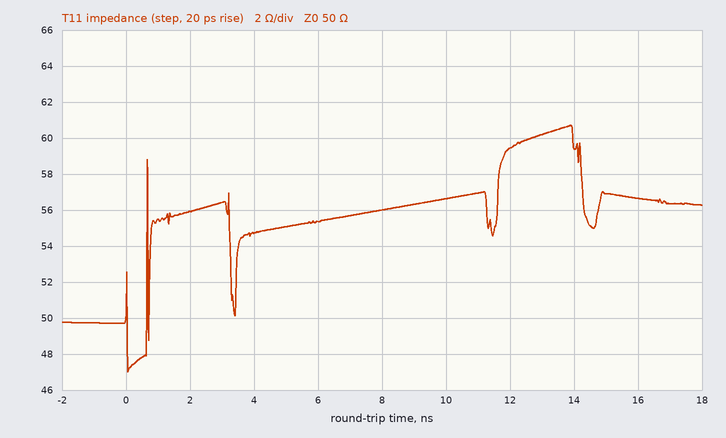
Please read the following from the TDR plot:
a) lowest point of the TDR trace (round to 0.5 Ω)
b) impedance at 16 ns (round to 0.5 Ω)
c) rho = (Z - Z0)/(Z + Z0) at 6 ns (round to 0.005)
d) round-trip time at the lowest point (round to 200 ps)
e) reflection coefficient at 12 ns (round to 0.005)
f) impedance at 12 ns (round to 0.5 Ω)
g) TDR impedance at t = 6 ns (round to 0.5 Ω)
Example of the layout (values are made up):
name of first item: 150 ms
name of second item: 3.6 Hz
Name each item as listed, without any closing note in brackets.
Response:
lowest point of the TDR trace: 47.0 Ω
impedance at 16 ns: 56.5 Ω
rho = (Z - Z0)/(Z + Z0) at 6 ns: +0.050
round-trip time at the lowest point: 0.0 ns
reflection coefficient at 12 ns: +0.085
impedance at 12 ns: 59.5 Ω
TDR impedance at t = 6 ns: 55.5 Ω
